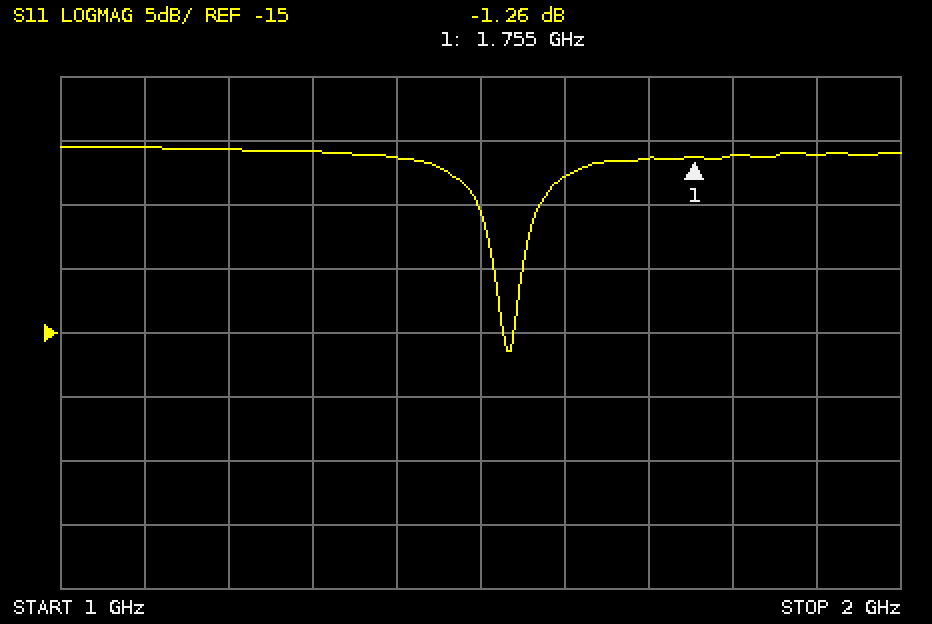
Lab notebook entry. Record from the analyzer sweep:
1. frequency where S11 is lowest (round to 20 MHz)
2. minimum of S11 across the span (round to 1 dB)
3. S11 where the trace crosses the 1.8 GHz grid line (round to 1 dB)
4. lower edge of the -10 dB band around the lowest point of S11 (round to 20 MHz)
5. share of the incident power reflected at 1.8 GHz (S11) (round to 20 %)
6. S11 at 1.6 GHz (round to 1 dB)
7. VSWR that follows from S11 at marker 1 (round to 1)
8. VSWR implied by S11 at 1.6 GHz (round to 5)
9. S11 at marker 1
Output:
1.54 GHz
-16 dB
-1 dB
1.52 GHz
80 %
-3 dB
14
5
-1.26 dB
